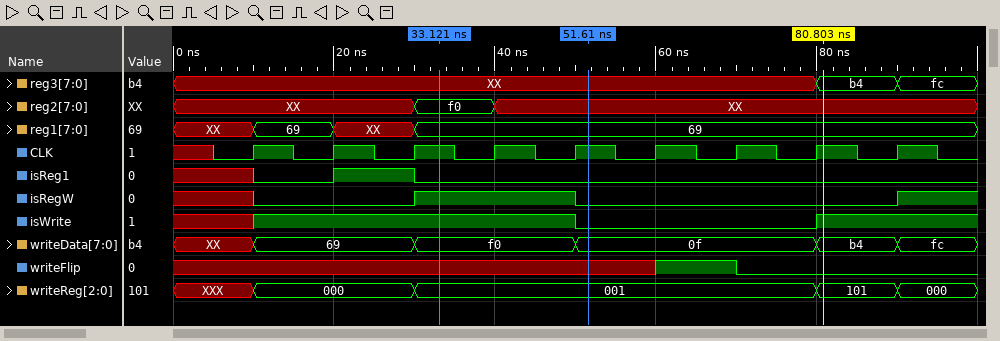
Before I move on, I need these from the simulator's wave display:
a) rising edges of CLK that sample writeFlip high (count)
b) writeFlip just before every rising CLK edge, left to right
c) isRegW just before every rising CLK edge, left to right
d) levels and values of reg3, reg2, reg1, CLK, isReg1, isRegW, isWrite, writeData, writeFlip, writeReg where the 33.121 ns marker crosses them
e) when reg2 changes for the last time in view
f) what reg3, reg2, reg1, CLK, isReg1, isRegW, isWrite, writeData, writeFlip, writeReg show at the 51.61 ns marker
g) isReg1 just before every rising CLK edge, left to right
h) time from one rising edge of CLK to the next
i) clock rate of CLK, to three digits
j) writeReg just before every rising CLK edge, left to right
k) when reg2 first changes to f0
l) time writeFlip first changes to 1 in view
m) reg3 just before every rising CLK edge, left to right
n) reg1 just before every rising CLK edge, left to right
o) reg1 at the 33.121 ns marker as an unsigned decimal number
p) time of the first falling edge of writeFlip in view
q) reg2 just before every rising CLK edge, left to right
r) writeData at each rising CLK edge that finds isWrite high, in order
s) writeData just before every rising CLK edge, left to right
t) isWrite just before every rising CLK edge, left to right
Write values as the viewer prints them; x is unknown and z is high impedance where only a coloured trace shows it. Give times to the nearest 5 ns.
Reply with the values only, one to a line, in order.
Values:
1
x x x x x x 1 0 0
x 0 0 1 1 0 0 0 0
reg3=XX, reg2=f0, reg1=69, CLK=1, isReg1=0, isRegW=1, isWrite=1, writeData=f0, writeFlip=x, writeReg=001
40 ns
reg3=XX, reg2=XX, reg1=69, CLK=1, isReg1=0, isRegW=0, isWrite=0, writeData=0f, writeFlip=x, writeReg=001
x 0 1 0 0 0 0 0 0
10 ns
100 MHz
XXX, 000, 000, 001, 001, 001, 001, 001, 101
30 ns
60 ns
XX, XX, XX, XX, XX, XX, XX, XX, b4
XX, 69, XX, 69, 69, 69, 69, 69, 69
105
70 ns
XX, XX, XX, f0, XX, XX, XX, XX, XX
69, 69, f0, f0, b4
XX, 69, 69, f0, f0, 0f, 0f, 0f, b4
x 1 1 1 1 0 0 0 1
